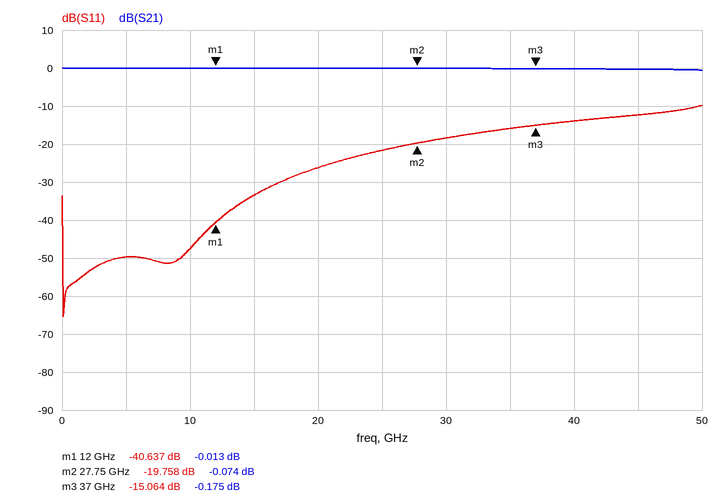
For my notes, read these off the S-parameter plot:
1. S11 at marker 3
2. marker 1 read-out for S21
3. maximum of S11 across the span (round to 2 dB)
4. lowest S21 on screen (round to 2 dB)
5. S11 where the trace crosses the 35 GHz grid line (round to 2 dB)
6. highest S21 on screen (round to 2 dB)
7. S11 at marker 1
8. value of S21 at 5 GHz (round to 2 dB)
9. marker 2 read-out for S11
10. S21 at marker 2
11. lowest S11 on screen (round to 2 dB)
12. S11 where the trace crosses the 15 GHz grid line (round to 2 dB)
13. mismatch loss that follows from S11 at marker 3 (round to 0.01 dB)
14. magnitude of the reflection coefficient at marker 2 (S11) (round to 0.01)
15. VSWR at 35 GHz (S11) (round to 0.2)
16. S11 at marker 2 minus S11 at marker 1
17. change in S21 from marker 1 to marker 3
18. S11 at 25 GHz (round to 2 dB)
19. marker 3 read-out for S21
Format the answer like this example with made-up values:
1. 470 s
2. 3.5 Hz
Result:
1. -15.064 dB
2. -0.013 dB
3. -10 dB
4. 0 dB
5. -16 dB
6. 0 dB
7. -40.637 dB
8. 0 dB
9. -19.758 dB
10. -0.074 dB
11. -66 dB
12. -34 dB
13. 0.14 dB
14. 0.10
15. 1.4
16. 20.879 dB
17. -0.162 dB
18. -22 dB
19. -0.175 dB
